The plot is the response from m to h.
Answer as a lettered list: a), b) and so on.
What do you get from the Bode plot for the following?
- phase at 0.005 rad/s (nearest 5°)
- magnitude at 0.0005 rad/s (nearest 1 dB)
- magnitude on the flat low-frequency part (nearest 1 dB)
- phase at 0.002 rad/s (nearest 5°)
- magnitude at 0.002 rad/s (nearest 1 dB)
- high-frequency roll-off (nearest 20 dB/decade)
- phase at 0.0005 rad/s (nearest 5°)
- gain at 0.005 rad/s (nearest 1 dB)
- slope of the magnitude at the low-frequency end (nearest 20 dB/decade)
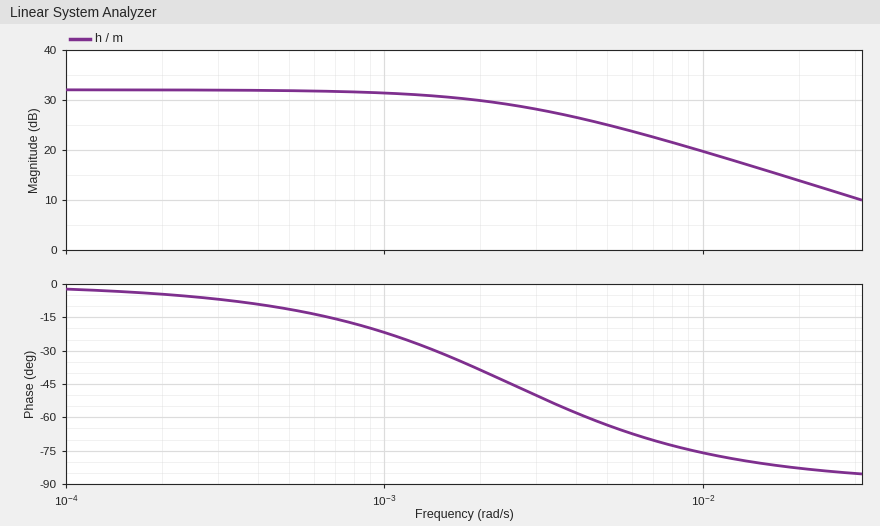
a) -65°
b) 32 dB
c) 32 dB
d) -40°
e) 30 dB
f) -20 dB/decade
g) -10°
h) 25 dB
i) 0 dB/decade
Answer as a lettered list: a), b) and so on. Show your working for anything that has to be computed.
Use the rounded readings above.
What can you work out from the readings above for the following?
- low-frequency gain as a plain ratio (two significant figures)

a) 10^(32 / 20) = 40
